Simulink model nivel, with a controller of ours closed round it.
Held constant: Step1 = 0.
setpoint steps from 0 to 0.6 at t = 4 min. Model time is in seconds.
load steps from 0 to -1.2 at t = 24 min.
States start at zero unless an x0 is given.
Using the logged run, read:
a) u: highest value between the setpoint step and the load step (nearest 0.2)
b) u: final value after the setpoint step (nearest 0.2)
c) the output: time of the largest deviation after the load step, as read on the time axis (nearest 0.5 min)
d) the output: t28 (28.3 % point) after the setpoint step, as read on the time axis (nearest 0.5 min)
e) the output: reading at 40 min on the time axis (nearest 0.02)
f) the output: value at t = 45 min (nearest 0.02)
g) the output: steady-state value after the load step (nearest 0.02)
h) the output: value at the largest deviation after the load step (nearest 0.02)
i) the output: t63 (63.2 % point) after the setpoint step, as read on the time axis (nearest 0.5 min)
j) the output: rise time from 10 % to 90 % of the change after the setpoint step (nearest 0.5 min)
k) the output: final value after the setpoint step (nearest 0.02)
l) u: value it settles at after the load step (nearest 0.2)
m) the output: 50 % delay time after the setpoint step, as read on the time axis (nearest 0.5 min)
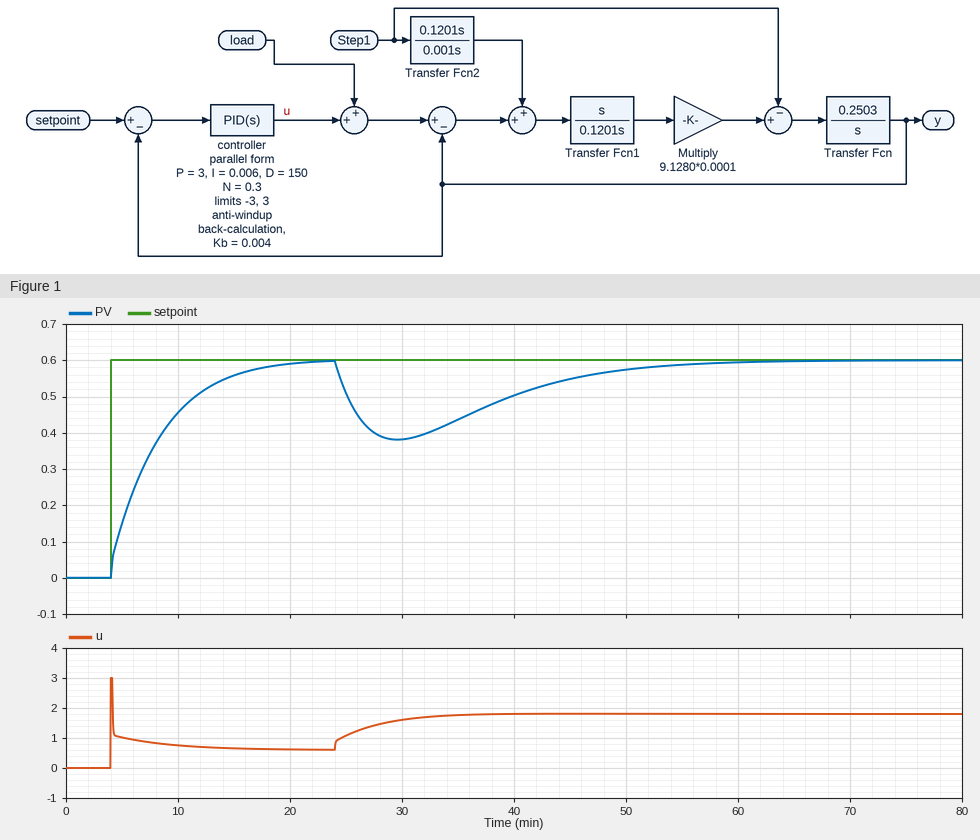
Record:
3.0
0.6
29.5 min
5.0 min
0.50
0.54
0.60
0.38
8.0 min
9.5 min
0.60
1.8
7.0 min
